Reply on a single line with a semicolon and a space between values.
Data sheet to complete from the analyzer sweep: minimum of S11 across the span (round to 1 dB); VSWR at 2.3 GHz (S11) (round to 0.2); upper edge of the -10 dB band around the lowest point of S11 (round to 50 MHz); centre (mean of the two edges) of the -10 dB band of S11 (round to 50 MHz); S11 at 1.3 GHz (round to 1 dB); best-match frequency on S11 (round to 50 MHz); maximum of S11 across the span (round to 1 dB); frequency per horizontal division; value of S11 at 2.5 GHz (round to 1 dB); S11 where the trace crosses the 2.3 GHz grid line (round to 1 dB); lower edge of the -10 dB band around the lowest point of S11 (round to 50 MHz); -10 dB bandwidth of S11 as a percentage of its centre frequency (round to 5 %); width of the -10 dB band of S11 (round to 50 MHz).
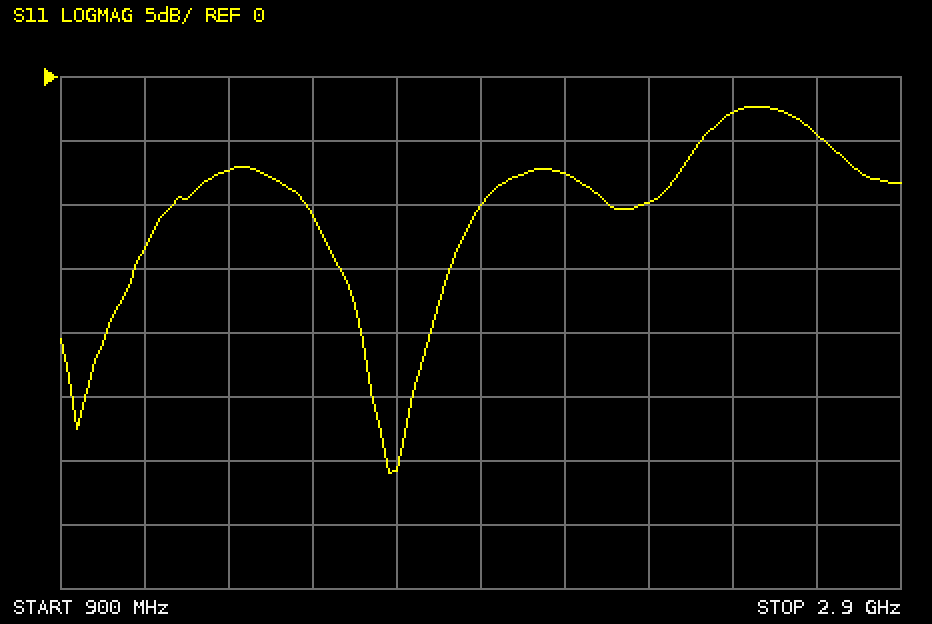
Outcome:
-31 dB; 2.0; 1.90 GHz; 1.70 GHz; -7 dB; 1.70 GHz; -2 dB; 200 MHz; -3 dB; -10 dB; 1.50 GHz; 25 %; 400 MHz
